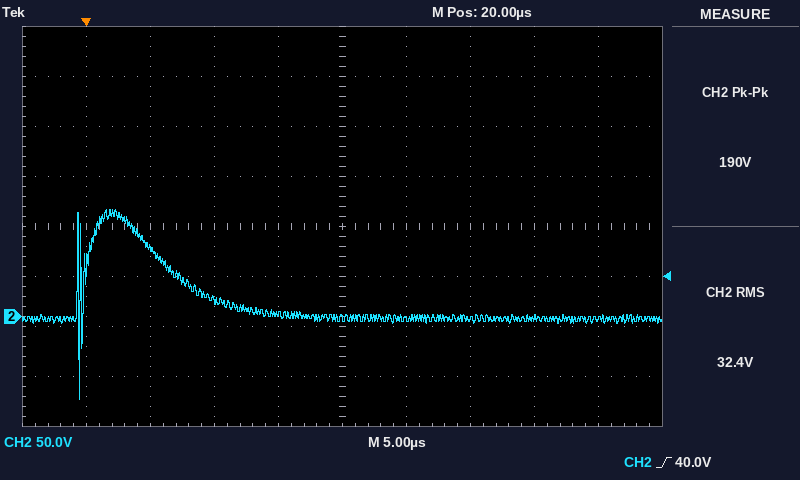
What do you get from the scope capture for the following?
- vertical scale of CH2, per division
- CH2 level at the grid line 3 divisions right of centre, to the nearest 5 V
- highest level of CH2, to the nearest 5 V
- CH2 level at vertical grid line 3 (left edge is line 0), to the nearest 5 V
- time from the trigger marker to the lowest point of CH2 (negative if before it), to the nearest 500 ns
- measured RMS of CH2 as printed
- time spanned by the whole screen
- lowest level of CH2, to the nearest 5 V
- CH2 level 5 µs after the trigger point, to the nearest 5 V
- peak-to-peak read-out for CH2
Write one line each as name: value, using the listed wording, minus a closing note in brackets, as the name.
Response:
vertical scale of CH2, per division: 50 V
CH2 level at the grid line 3 divisions right of centre, to the nearest 5 V: 0 V
highest level of CH2, to the nearest 5 V: 105 V
CH2 level at vertical grid line 3 (left edge is line 0), to the nearest 5 V: 15 V
time from the trigger marker to the lowest point of CH2 (negative if before it), to the nearest 500 ns: -500 ns
measured RMS of CH2 as printed: 32.4 V
time spanned by the whole screen: 50 µs
lowest level of CH2, to the nearest 5 V: -85 V
CH2 level 5 µs after the trigger point, to the nearest 5 V: 70 V
peak-to-peak read-out for CH2: 190 V
